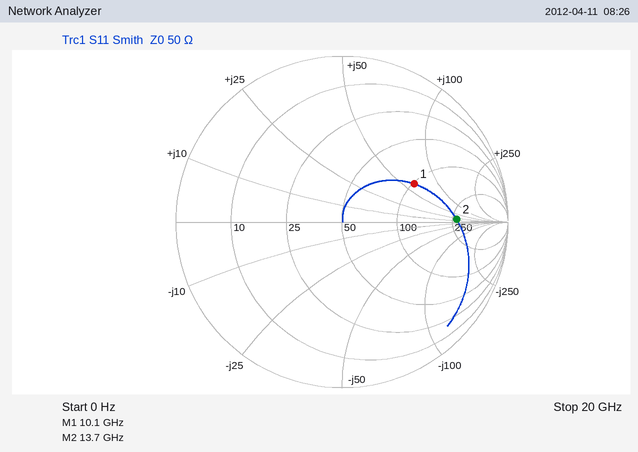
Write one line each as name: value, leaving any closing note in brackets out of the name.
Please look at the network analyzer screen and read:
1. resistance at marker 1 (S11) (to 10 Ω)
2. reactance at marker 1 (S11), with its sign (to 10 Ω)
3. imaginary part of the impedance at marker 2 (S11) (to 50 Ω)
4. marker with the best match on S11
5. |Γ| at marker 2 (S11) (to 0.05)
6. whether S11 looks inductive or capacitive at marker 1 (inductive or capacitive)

resistance at marker 1 (S11): 100 Ω
reactance at marker 1 (S11), with its sign: +60 Ω
imaginary part of the impedance at marker 2 (S11): 0 Ω
marker with the best match on S11: marker 1
|Γ| at marker 2 (S11): 0.70
whether S11 looks inductive or capacitive at marker 1: inductive
